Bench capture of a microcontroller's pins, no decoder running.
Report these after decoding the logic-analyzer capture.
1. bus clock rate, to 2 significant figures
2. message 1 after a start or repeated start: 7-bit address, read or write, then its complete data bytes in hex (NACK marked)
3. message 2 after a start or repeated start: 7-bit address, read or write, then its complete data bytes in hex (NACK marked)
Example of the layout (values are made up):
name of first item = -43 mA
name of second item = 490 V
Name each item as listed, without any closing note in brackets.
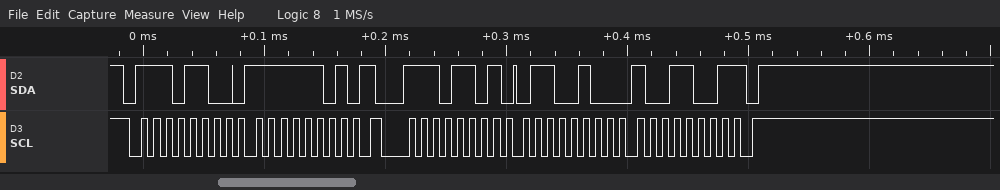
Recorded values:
bus clock rate, to 2 significant figures = 100 kHz
message 1 after a start or repeated start: 7-bit address, read or write, then its complete data bytes in hex = 0x76 write: FD
message 2 after a start or repeated start: 7-bit address, read or write, then its complete data bytes in hex = 0x76 read: 64 99 NACK
